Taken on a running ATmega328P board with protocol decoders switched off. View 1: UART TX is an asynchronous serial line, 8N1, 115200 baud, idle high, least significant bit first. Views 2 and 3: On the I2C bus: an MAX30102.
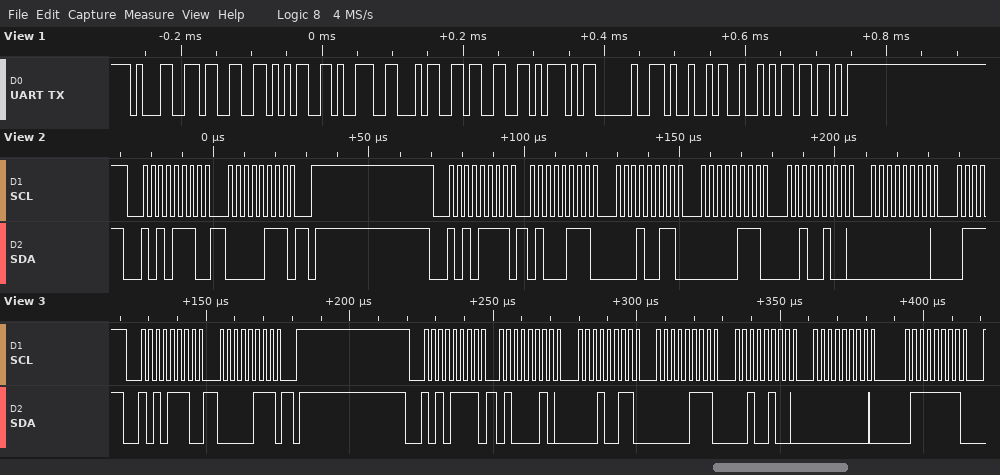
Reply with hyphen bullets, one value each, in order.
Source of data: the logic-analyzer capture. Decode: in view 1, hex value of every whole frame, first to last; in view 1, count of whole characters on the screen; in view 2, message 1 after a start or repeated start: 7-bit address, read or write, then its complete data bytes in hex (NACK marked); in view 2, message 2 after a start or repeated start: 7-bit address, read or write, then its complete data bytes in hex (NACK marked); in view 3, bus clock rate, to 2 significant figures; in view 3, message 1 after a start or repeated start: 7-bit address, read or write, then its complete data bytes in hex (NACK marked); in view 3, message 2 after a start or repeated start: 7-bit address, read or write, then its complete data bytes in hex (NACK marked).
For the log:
- 31 33 35 39 34 33 5D 20 49 52 5B
- 11
- 0x57 write: 07
- 0x57 read: 47 13 07 24 00
- 400 kHz
- 0x57 write: 07
- 0x57 read: 42 13 07 24 00 7F
